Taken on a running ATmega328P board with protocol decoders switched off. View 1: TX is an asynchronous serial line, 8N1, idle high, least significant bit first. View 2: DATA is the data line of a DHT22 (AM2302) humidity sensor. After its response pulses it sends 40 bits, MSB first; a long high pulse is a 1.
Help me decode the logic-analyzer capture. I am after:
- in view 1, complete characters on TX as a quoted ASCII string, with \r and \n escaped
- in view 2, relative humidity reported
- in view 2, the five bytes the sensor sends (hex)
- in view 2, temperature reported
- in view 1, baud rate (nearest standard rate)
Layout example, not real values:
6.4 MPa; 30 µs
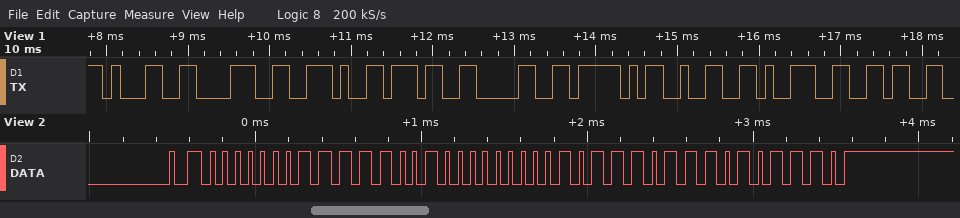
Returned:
"18.70_296"; 49.8 %; 01 F2 00 BB AE; 18.7 °C; 9600 baud
